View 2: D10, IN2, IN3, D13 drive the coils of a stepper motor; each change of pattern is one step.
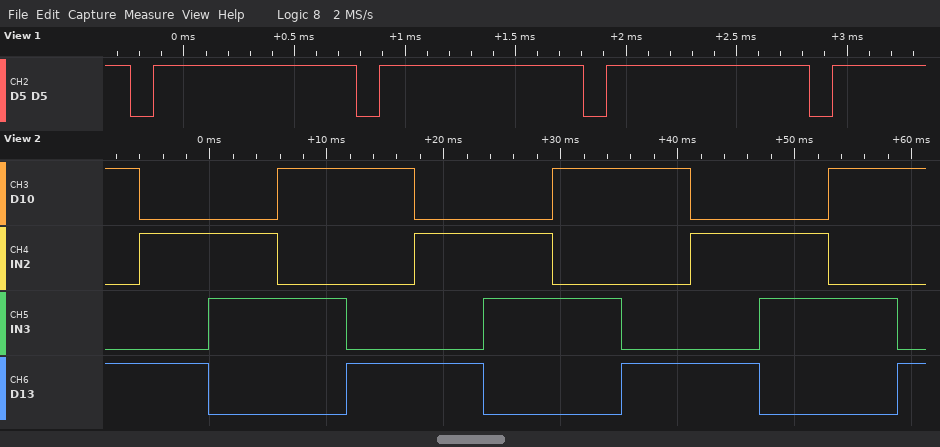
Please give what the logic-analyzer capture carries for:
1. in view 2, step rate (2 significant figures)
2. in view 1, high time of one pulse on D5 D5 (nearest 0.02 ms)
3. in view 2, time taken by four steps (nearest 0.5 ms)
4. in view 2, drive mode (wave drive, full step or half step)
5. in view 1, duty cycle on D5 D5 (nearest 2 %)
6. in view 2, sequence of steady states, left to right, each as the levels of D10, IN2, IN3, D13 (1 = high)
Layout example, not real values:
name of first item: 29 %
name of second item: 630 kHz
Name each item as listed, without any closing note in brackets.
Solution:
in view 2, step rate: 170 steps/s
in view 1, high time of one pulse on D5 D5: 0.92 ms
in view 2, time taken by four steps: 23.5 ms
in view 2, drive mode: full step
in view 1, duty cycle on D5 D5: 90 %
in view 2, sequence of steady states, left to right, each as the levels of D10, IN2, IN3, D13: 1001 0101 0110 1010 1001 0101 0110 1010 1001 0101 0110 1010 1001
